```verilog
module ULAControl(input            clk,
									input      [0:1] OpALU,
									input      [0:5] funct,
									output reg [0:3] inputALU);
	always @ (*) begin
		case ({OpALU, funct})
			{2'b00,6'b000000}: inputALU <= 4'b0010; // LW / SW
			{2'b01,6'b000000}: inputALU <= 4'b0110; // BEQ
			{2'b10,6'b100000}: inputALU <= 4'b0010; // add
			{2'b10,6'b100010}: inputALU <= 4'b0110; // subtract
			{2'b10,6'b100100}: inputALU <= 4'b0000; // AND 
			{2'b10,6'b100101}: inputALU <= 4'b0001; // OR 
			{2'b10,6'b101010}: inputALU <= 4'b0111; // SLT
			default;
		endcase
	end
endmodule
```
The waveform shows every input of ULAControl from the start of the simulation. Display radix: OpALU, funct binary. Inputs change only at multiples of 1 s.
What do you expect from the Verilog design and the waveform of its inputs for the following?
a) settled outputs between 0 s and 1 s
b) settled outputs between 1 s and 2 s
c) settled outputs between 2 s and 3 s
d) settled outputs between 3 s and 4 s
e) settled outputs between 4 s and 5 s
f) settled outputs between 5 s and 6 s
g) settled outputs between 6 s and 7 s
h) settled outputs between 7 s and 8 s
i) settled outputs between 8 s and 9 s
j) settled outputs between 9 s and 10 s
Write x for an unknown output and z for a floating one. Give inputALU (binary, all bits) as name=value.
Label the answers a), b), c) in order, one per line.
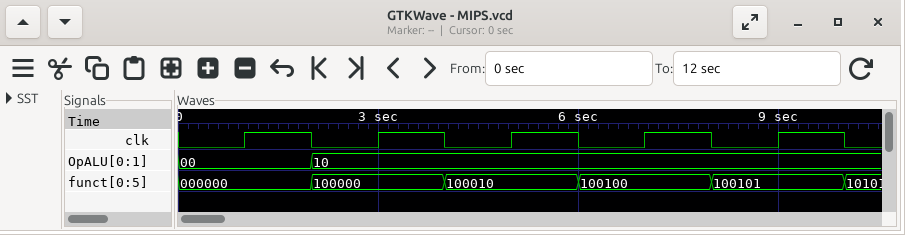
a) inputALU=0010
b) inputALU=0010
c) inputALU=0010
d) inputALU=0010
e) inputALU=0110
f) inputALU=0110
g) inputALU=0000
h) inputALU=0000
i) inputALU=0001
j) inputALU=0001
